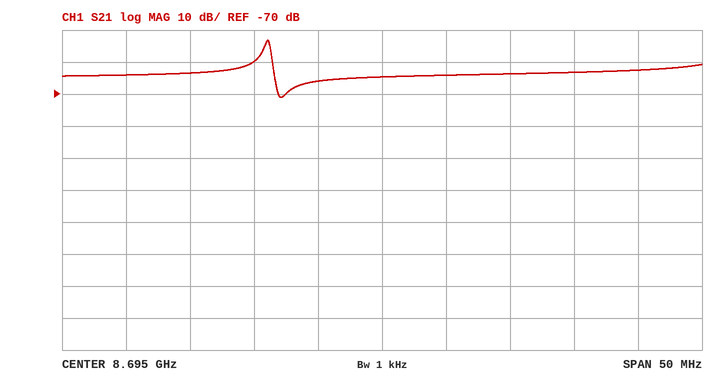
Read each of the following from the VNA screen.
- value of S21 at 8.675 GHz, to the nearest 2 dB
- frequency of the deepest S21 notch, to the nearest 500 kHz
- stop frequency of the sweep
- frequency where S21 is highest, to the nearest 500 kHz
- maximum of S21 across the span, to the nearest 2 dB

-64 dB
8.6870 GHz
8.72 GHz
8.6860 GHz
-54 dB
